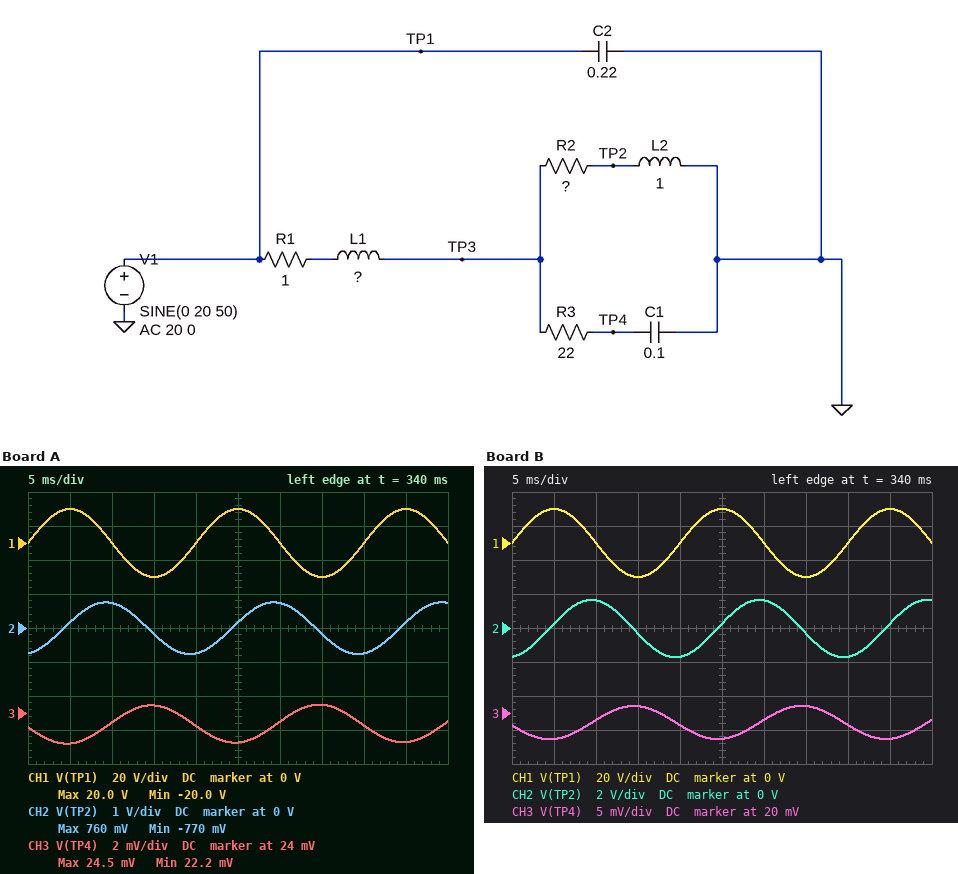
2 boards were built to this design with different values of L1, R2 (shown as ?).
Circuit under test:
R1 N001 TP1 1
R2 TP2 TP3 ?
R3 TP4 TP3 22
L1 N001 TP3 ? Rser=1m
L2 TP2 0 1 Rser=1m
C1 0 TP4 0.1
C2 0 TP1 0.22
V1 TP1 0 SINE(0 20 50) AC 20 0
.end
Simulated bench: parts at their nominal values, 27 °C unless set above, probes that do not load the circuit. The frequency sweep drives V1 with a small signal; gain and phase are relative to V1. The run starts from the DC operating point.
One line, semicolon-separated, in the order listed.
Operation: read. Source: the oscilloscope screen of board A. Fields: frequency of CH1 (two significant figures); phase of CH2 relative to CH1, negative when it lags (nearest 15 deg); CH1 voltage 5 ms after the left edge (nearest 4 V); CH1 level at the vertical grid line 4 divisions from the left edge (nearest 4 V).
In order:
50 Hz; -75 deg; 20 V; 0 V
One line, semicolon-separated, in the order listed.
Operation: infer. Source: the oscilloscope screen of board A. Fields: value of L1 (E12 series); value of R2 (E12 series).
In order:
1.8 H; 39 Ω
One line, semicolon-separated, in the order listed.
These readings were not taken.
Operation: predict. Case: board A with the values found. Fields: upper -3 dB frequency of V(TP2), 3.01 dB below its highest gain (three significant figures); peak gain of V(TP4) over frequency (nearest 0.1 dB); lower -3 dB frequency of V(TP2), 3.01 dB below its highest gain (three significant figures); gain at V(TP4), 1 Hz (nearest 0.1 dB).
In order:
12.7 Hz; -0.2 dB; 987 mHz; -25.4 dB
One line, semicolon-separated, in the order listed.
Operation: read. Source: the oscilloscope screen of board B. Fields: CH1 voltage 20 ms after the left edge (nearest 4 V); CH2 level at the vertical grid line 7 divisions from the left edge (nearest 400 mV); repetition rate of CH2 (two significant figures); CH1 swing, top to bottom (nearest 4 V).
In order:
0 V; -400 mV; 50 Hz; 40 V
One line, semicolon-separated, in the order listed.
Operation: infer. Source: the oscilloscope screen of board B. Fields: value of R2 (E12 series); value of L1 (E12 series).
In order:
5.6 Ω; 820 mH
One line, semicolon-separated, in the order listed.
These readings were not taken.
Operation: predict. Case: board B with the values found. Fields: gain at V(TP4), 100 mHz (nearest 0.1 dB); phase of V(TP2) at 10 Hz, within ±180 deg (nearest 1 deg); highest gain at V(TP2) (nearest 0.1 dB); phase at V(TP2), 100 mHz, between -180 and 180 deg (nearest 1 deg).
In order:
-6.3 dB; -47 deg; -6.3 dB; 78 deg
